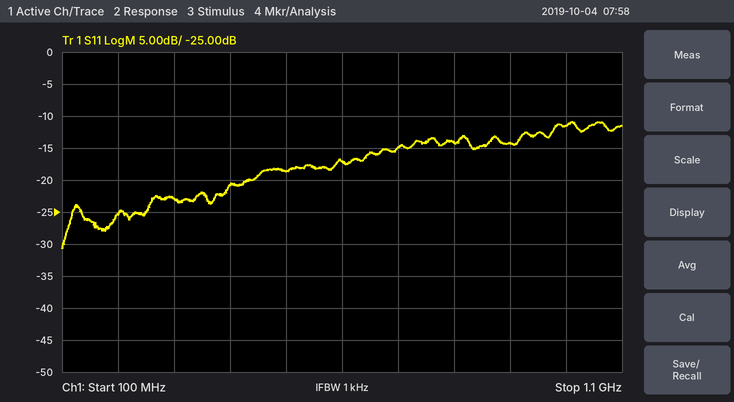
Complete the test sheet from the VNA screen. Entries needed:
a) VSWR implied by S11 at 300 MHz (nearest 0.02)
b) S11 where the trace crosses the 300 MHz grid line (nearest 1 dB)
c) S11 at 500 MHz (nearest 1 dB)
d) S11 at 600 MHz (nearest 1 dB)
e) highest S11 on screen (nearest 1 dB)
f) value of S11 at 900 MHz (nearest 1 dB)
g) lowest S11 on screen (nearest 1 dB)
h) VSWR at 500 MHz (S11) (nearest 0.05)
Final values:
1.16
-23 dB
-19 dB
-17 dB
-11 dB
-14 dB
-31 dB
1.25
